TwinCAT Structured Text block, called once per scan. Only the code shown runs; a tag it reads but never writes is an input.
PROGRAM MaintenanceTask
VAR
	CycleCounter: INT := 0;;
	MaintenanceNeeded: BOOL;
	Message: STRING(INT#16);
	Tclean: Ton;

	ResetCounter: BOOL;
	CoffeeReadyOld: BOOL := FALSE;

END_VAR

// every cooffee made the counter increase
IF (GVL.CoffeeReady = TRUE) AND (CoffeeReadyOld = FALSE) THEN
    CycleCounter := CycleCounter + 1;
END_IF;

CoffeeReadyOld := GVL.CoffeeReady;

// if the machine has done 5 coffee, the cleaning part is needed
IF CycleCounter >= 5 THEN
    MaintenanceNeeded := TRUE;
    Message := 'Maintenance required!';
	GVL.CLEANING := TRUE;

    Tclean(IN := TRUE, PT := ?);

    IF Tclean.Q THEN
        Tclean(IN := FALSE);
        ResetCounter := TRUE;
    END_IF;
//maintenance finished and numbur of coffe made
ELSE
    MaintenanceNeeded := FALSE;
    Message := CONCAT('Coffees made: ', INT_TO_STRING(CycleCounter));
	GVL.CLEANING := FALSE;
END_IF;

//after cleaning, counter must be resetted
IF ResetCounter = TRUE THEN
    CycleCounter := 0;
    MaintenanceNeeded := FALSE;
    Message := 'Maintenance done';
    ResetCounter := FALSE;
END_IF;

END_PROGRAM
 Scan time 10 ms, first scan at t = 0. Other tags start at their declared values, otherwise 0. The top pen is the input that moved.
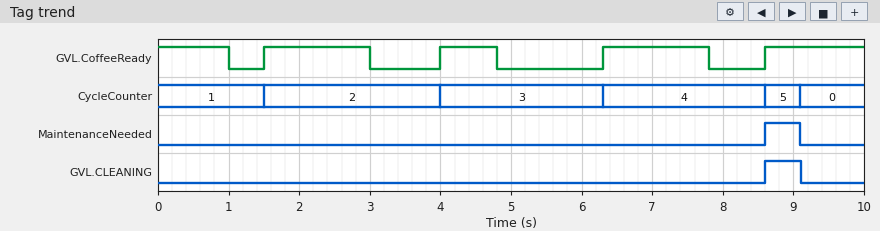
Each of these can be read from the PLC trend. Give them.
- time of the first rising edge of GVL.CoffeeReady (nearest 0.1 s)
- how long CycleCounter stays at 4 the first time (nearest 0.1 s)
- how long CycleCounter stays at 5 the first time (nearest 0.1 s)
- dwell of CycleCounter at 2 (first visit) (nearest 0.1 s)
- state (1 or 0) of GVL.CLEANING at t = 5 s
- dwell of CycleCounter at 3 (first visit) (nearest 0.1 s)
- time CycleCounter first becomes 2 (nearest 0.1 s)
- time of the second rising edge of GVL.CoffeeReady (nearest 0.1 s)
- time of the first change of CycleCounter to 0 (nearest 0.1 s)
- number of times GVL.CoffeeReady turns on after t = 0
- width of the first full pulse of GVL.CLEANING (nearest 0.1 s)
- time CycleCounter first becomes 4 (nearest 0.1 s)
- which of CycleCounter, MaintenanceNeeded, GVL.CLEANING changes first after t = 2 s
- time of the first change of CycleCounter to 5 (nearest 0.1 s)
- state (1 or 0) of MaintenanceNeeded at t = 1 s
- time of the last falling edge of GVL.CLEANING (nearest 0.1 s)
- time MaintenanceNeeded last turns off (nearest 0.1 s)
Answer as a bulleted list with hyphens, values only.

- 1.5 s
- 2.3 s
- 0.5 s
- 2.5 s
- 0
- 2.3 s
- 1.5 s
- 4.0 s
- 9.1 s
- 4
- 0.5 s
- 6.3 s
- CycleCounter
- 8.6 s
- 0
- 9.1 s
- 9.1 s
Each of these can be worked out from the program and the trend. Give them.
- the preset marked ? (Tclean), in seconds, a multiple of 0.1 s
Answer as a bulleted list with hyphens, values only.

- 0.5 s
